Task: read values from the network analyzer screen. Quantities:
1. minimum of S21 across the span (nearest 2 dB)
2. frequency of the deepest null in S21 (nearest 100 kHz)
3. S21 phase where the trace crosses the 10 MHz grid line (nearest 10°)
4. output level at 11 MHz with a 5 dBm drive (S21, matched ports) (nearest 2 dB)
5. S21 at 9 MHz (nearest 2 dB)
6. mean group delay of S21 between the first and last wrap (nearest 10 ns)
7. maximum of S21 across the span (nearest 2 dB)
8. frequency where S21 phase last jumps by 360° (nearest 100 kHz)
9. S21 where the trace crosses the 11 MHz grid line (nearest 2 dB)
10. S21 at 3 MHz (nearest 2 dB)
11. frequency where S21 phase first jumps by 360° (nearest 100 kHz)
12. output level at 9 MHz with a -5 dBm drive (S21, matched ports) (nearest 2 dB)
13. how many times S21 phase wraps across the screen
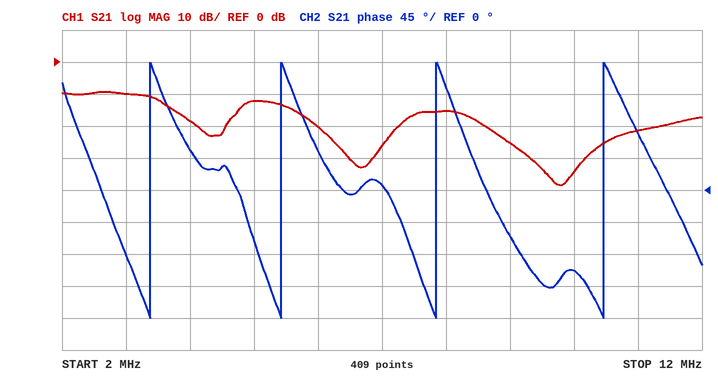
-38 dB
9.8 MHz
-110°
-16 dBm
-26 dB
420 ns
-10 dB
10.5 MHz
-22 dB
-10 dB
3.4 MHz
-30 dBm
4
